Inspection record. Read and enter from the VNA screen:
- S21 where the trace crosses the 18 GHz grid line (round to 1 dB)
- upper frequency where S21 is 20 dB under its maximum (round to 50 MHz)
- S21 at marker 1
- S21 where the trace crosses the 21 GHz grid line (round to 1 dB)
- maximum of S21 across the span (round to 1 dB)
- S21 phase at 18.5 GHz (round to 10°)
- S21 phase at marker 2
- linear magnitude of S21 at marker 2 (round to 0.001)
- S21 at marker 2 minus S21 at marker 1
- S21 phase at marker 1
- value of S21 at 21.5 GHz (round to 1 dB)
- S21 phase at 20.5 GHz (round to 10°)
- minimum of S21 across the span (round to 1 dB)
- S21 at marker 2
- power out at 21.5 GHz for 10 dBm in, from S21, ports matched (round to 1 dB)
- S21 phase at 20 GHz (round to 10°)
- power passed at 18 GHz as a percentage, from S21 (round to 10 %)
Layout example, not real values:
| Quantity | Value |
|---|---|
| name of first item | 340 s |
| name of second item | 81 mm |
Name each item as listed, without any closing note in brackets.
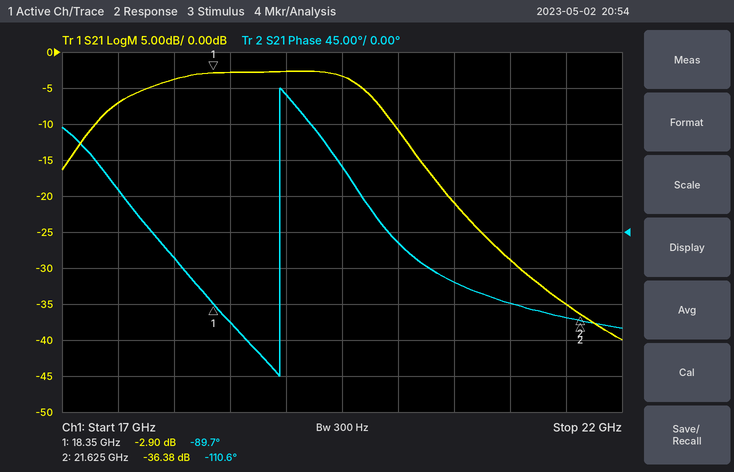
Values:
| Quantity | Value |
|---|---|
| S21 where the trace crosses the 18 GHz grid line | -4 dB |
| upper frequency where S21 is 20 dB under its maximum | 20.60 GHz |
| S21 at marker 1 | -2.90 dB |
| S21 where the trace crosses the 21 GHz grid line | -29 dB |
| maximum of S21 across the span | -3 dB |
| S21 phase at 18.5 GHz | -110° |
| S21 phase at marker 2 | -110.6° |
| linear magnitude of S21 at marker 2 | 0.015 |
| S21 at marker 2 minus S21 at marker 1 | -33.48 dB |
| S21 phase at marker 1 | -89.7° |
| value of S21 at 21.5 GHz | -35 dB |
| S21 phase at 20.5 GHz | -60° |
| minimum of S21 across the span | -40 dB |
| S21 at marker 2 | -36.38 dB |
| power out at 21.5 GHz for 10 dBm in, from S21, ports matched | -25 dBm |
| S21 phase at 20 GHz | -10° |
| power passed at 18 GHz as a percentage, from S21 | 40 % |
